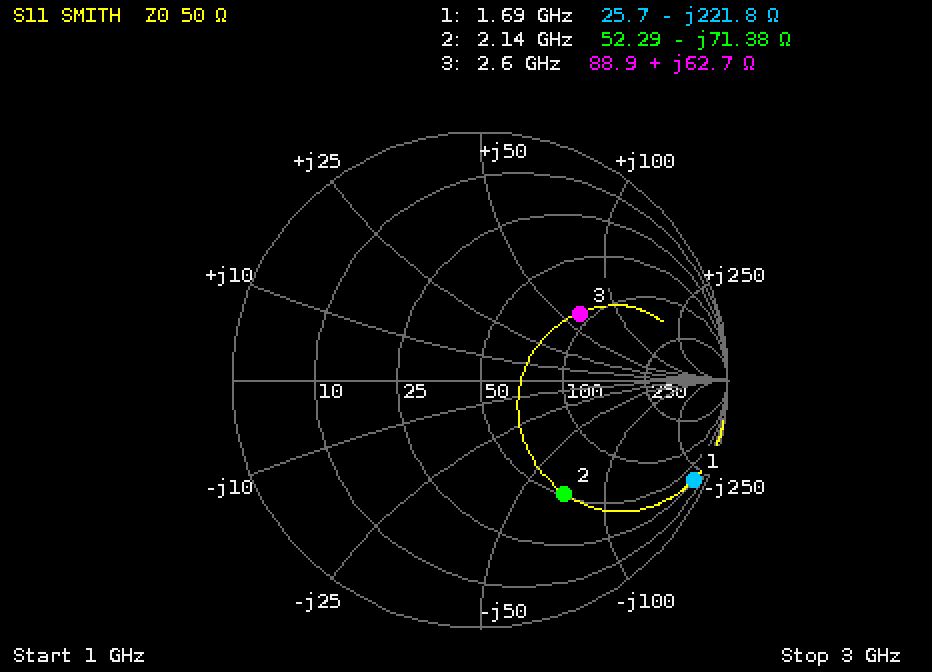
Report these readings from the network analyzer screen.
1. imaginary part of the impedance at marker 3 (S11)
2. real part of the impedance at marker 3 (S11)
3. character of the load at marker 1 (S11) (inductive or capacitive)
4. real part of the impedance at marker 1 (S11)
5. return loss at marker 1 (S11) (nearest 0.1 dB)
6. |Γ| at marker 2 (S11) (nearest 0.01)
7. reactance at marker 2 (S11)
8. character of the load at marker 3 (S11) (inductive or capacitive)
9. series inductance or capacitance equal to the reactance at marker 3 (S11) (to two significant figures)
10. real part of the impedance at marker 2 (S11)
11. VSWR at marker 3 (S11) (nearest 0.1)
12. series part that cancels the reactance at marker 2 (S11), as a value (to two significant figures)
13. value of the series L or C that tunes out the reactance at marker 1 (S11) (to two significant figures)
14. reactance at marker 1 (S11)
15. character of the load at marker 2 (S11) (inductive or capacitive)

+62.7 Ω
88.9 Ω
capacitive
25.7 Ω
0.4 dB
0.57
-71.38 Ω
inductive
3.8 nH
52.29 Ω
2.9
5.3 nH
21 nH
-221.8 Ω
capacitive
